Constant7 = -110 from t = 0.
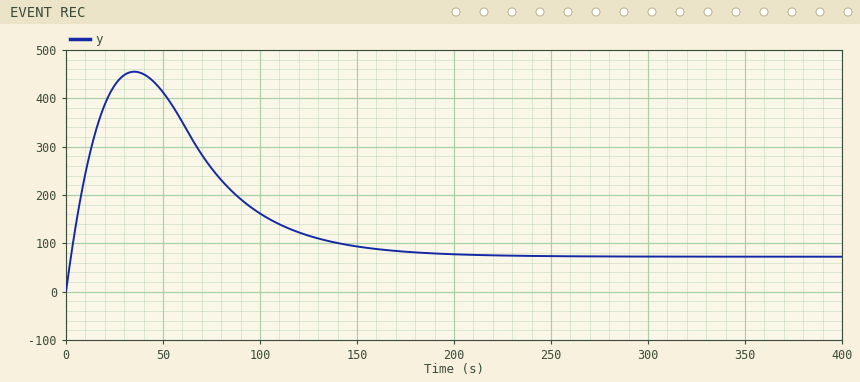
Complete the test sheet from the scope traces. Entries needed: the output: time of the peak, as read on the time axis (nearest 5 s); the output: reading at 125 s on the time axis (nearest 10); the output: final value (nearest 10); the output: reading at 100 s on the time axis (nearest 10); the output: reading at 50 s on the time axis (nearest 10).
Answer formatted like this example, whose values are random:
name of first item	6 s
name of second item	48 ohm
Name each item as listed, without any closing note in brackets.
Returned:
the output: time of the peak, as read on the time axis	35 s
the output: reading at 125 s on the time axis	120
the output: final value	70
the output: reading at 100 s on the time axis	160
the output: reading at 50 s on the time axis	410
